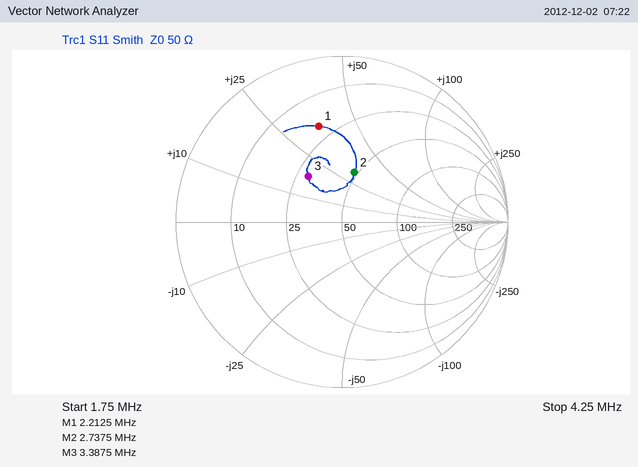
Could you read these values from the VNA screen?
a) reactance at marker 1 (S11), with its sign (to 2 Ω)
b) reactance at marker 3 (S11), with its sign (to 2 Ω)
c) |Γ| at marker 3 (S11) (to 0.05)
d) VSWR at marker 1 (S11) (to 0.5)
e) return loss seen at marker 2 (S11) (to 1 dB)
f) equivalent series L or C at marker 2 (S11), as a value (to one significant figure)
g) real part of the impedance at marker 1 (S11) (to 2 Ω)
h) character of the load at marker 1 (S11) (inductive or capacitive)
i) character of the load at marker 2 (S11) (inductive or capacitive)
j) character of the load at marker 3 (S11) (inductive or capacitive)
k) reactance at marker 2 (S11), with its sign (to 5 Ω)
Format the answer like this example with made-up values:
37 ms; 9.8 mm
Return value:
+36 Ω; +18 Ω; 0.35; 4.0; 10 dB; 2 µH; 20 Ω; inductive; inductive; inductive; +30 Ω
